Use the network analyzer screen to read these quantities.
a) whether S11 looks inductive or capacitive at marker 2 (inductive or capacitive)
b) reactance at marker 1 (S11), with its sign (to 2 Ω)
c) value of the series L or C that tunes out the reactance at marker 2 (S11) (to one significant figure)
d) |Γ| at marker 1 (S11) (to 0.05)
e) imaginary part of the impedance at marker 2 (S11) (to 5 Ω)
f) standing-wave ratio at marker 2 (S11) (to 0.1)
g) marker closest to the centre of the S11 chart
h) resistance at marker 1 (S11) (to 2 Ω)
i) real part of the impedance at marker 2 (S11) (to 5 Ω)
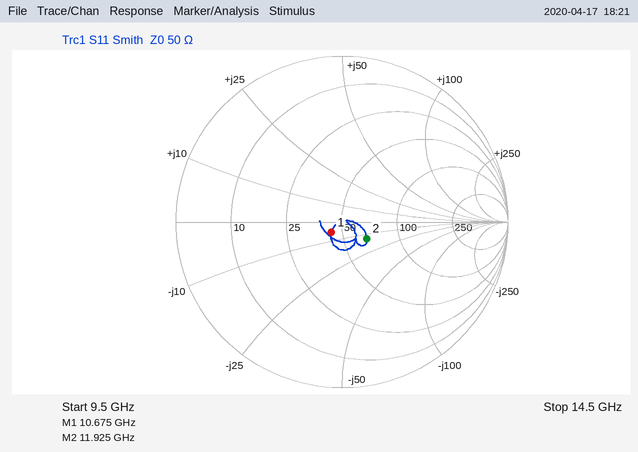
capacitive
-6 Ω
200 pH
0.10
-15 Ω
1.4
marker 1
44 Ω
65 Ω
